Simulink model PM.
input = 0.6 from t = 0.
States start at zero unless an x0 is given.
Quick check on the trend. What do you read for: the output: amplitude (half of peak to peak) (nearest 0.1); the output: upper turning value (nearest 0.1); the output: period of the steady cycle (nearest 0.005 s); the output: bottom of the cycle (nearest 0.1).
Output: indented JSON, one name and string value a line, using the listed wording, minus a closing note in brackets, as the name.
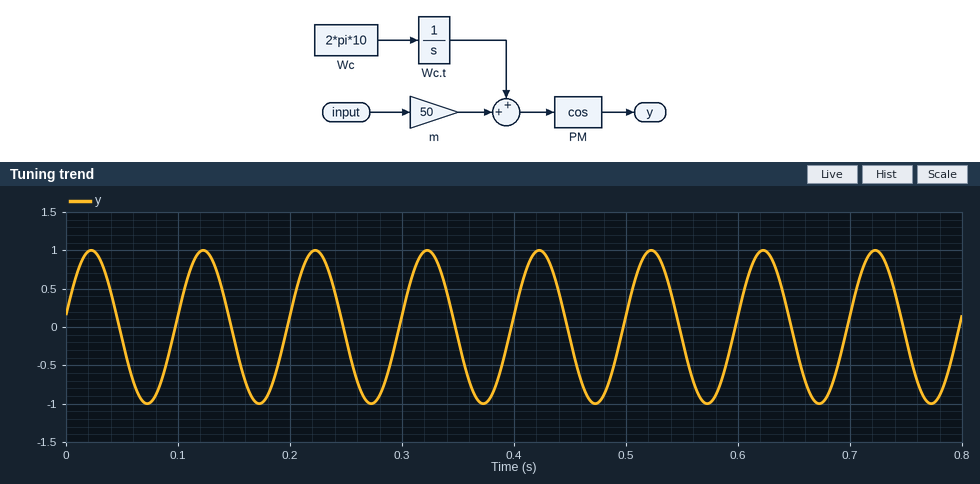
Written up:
{
  "the output: amplitude (half of peak to peak)": "1.0",
  "the output: upper turning value": "1.0",
  "the output: period of the steady cycle": "0.100 s",
  "the output: bottom of the cycle": "-1.0"
}
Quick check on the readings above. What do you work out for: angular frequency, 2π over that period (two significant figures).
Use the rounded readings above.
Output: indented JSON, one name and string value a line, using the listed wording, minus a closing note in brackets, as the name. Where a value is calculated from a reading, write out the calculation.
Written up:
{
  "angular frequency, 2π over that period": "2π / 0.1 = 63 rad/s"
}
